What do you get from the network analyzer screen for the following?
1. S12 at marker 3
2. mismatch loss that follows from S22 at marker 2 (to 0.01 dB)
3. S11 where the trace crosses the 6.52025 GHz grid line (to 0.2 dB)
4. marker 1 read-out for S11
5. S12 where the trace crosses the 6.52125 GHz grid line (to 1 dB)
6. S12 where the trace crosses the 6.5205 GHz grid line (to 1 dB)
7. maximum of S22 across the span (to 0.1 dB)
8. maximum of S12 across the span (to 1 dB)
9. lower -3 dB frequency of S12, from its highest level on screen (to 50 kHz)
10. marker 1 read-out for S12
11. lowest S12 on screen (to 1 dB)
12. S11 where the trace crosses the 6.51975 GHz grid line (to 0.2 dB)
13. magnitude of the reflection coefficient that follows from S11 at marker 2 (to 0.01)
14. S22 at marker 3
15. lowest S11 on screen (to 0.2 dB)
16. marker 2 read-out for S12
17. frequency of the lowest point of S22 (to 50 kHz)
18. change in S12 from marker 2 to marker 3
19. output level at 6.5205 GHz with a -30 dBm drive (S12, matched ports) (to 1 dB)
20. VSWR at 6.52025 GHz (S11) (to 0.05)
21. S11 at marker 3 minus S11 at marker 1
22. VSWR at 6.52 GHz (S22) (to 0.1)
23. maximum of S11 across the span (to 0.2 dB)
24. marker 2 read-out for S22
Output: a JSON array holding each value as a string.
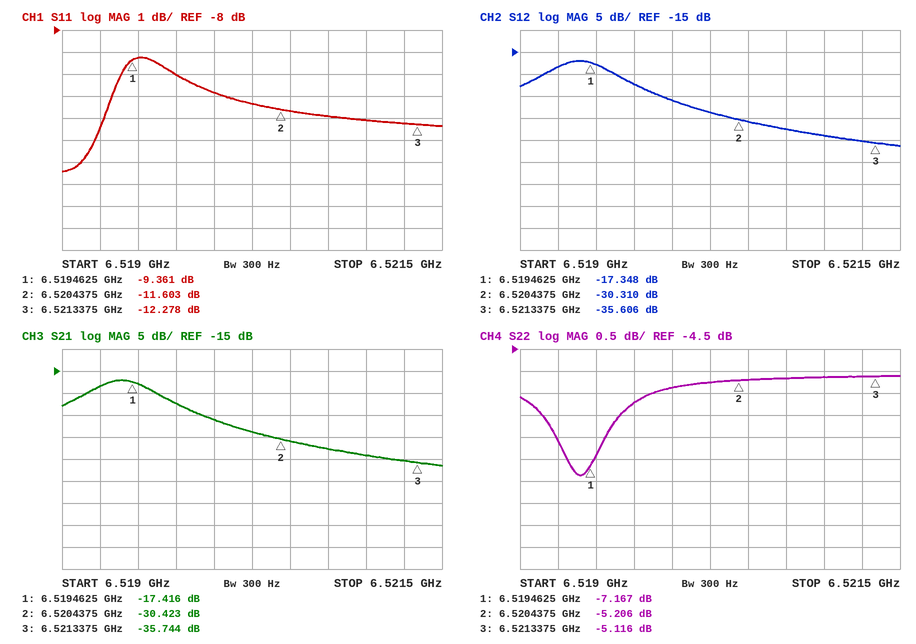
["-35.606 dB", "1.56 dB", "-11.4 dB", "-9.361 dB", "-35 dB", "-31 dB", "-5.1 dB", "-17 dB", "6.51915 GHz", "-17.348 dB", "-36 dB", "-10.0 dB", "0.26", "-5.116 dB", "-14.4 dB", "-30.310 dB", "6.51940 GHz", "-5.296 dB", "-61 dBm", "1.75", "-2.917 dB", "3.3", "-9.2 dB", "-5.206 dB"]
